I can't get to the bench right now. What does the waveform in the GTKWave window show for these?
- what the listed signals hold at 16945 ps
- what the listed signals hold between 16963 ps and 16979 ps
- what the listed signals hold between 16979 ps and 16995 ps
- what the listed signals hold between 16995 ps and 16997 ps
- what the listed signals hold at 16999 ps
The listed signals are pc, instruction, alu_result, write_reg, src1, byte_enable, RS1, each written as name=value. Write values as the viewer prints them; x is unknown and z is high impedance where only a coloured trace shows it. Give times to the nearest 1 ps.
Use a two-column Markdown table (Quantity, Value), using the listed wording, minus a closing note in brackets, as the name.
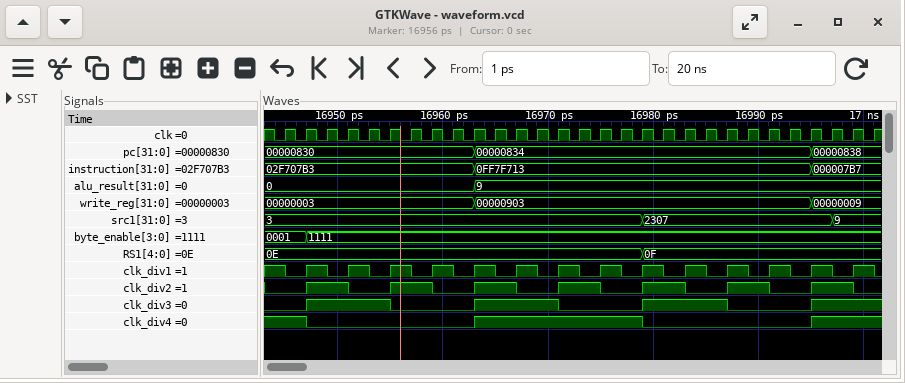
| Quantity | Value |
|---|---|
| what the listed signals hold at 16945 ps | pc=00000830, instruction=02F707B3, alu_result=0, write_reg=00000003, src1=3, byte_enable=0001, RS1=0E |
| what the listed signals hold between 16963 ps and 16979 ps | pc=00000834, instruction=0FF7F713, alu_result=9, write_reg=00000903, src1=3, byte_enable=1111, RS1=0E |
| what the listed signals hold between 16979 ps and 16995 ps | pc=00000834, instruction=0FF7F713, alu_result=9, write_reg=00000903, src1=2307, byte_enable=1111, RS1=0F |
| what the listed signals hold between 16995 ps and 16997 ps | pc=00000838, instruction=000007B7, alu_result=9, write_reg=00000009, src1=2307, byte_enable=1111, RS1=0F |
| what the listed signals hold at 16999 ps | pc=00000838, instruction=000007B7, alu_result=9, write_reg=00000009, src1=9, byte_enable=1111, RS1=0F |
